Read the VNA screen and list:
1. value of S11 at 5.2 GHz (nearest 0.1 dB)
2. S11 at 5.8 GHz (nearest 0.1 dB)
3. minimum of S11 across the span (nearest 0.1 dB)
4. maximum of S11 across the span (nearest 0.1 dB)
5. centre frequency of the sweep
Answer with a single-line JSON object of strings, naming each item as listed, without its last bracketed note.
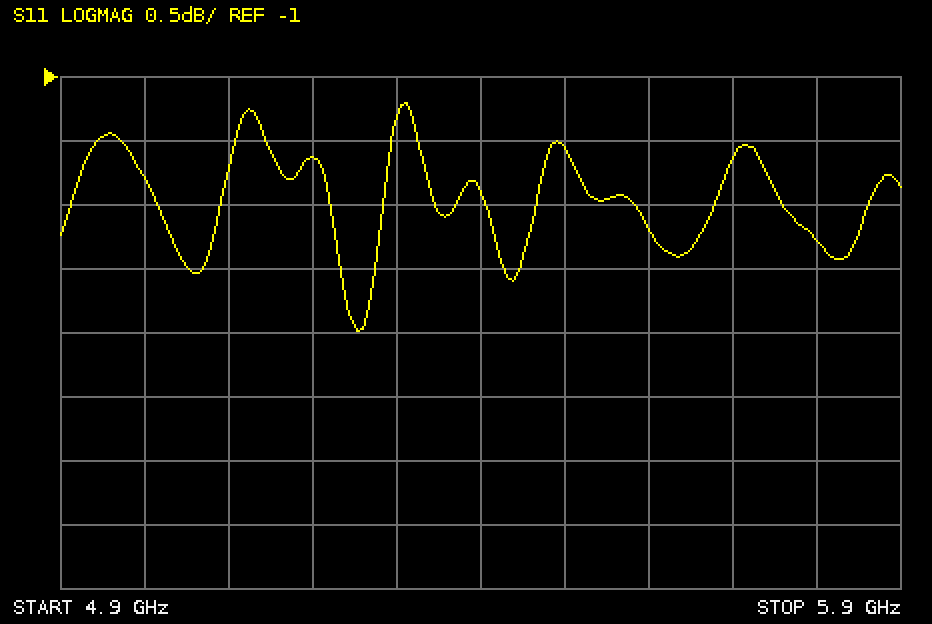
{"value of S11 at 5.2 GHz": "-1.6 dB", "S11 at 5.8 GHz": "-2.3 dB", "minimum of S11 across the span": "-3.0 dB", "maximum of S11 across the span": "-1.2 dB", "centre frequency of the sweep": "5.4 GHz"}
